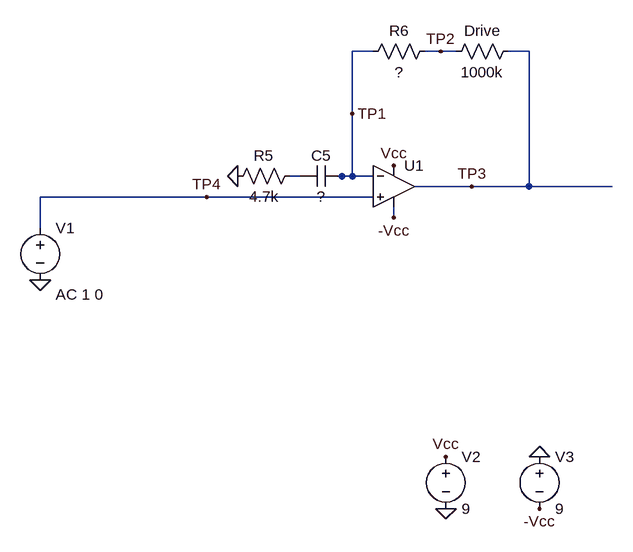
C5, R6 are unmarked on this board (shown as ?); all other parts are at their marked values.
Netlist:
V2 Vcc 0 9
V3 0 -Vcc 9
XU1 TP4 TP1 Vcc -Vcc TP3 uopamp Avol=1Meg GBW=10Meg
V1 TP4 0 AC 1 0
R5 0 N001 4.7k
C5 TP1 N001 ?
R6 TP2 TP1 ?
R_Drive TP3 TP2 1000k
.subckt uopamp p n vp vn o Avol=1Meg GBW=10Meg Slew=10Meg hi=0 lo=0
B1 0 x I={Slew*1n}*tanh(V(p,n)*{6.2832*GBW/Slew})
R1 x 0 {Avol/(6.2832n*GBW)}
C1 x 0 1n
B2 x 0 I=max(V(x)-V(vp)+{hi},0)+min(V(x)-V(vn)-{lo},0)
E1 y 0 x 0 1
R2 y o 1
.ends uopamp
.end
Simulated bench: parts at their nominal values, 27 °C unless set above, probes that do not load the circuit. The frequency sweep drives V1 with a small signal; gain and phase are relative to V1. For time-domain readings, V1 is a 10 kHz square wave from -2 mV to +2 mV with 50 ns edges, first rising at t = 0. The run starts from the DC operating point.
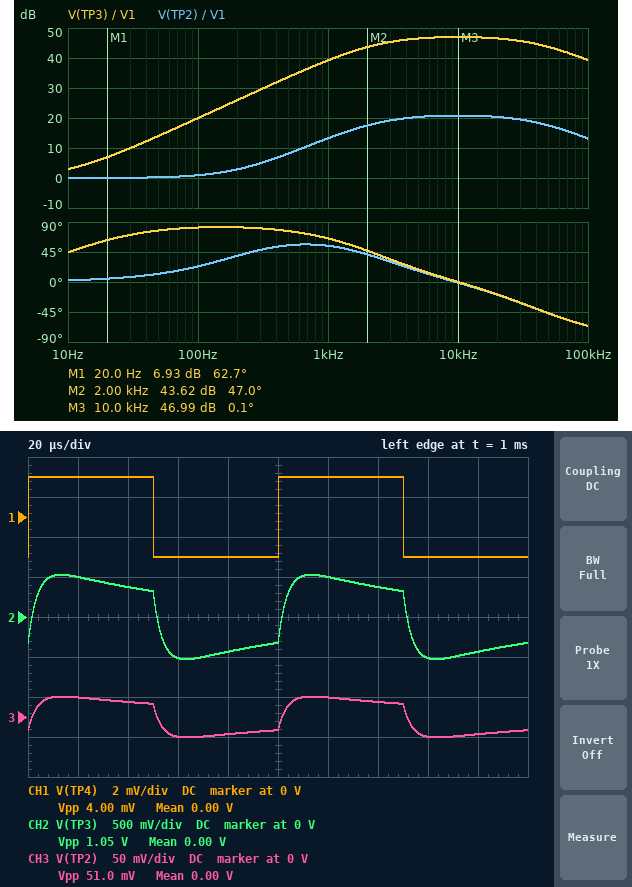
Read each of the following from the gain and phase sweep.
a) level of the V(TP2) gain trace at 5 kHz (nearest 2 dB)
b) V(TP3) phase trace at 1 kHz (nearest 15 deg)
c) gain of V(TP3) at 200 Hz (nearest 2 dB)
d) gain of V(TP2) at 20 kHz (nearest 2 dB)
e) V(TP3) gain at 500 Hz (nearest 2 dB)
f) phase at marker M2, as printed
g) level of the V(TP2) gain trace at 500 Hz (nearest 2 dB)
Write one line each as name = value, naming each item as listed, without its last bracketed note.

level of the V(TP2) gain trace at 5 kHz = 20 dB
V(TP3) phase trace at 1 kHz = 60 deg
gain of V(TP3) at 200 Hz = 26 dB
gain of V(TP2) at 20 kHz = 20 dB
V(TP3) gain at 500 Hz = 34 dB
phase at marker M2, as printed = 47.0 deg
level of the V(TP2) gain trace at 500 Hz = 8 dB
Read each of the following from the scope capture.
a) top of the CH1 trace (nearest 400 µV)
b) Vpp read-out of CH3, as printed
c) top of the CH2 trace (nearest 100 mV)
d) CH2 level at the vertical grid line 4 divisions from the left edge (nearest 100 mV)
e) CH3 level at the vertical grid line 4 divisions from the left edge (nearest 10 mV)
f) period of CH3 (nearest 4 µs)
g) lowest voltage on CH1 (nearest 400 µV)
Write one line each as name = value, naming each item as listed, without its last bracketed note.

top of the CH1 trace = 2.0 mV
Vpp read-out of CH3, as printed = 51.0 mV
top of the CH2 trace = 500 mV
CH2 level at the vertical grid line 4 divisions from the left edge = -400 mV
CH3 level at the vertical grid line 4 divisions from the left edge = -20 mV
period of CH3 = 100 µs
lowest voltage on CH1 = -2.0 mV
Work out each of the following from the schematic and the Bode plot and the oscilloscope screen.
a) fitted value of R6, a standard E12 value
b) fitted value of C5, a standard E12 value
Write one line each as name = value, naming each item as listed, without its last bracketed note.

fitted value of R6, a standard E12 value = 47 kΩ
fitted value of C5, a standard E12 value = 15 nF
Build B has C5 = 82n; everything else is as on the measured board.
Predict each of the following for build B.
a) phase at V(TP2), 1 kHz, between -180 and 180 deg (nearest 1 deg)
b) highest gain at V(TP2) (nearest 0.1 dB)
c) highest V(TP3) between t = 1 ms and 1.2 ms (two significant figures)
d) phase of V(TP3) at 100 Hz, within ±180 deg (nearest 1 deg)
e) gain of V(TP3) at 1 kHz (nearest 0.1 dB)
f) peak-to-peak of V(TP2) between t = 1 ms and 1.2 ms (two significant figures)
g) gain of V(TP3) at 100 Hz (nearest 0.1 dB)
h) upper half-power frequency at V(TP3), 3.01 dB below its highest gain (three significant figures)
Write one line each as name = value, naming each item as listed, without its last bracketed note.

phase at V(TP2), 1 kHz, between -180 and 180 deg = 19 deg
highest gain at V(TP2) = 20.8 dB
highest V(TP3) between t = 1 ms and 1.2 ms = 490 mV
phase of V(TP3) at 100 Hz, within ±180 deg = 75 deg
gain of V(TP3) at 1 kHz = 46.4 dB
peak-to-peak of V(TP2) between t = 1 ms and 1.2 ms = 45 mV
gain of V(TP3) at 100 Hz = 34.4 dB
upper half-power frequency at V(TP3), 3.01 dB below its highest gain = 45.1 kHz
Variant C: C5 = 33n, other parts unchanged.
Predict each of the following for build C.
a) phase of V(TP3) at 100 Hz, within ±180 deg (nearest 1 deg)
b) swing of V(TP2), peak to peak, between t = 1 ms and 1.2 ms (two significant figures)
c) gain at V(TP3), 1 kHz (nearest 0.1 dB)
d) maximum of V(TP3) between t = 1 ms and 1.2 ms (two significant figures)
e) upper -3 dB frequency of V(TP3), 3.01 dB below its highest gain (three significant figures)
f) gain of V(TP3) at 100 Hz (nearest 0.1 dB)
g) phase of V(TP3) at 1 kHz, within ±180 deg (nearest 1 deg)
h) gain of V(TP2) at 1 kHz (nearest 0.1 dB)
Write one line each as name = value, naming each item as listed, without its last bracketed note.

phase of V(TP3) at 100 Hz, within ±180 deg = 82 deg
swing of V(TP2), peak to peak, between t = 1 ms and 1.2 ms = 47 mV
gain at V(TP3), 1 kHz = 44.0 dB
maximum of V(TP3) between t = 1 ms and 1.2 ms = 480 mV
upper -3 dB frequency of V(TP3), 3.01 dB below its highest gain = 45.7 kHz
gain of V(TP3) at 100 Hz = 26.7 dB
phase of V(TP3) at 1 kHz, within ±180 deg = 45 deg
gain of V(TP2) at 1 kHz = 17.8 dB
